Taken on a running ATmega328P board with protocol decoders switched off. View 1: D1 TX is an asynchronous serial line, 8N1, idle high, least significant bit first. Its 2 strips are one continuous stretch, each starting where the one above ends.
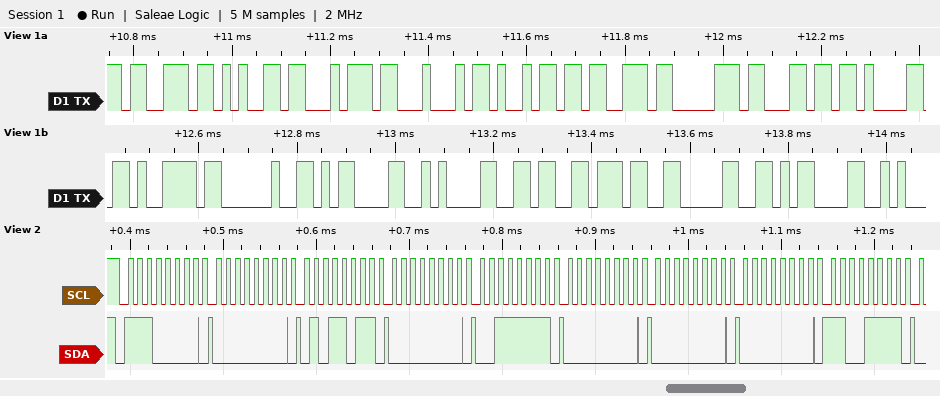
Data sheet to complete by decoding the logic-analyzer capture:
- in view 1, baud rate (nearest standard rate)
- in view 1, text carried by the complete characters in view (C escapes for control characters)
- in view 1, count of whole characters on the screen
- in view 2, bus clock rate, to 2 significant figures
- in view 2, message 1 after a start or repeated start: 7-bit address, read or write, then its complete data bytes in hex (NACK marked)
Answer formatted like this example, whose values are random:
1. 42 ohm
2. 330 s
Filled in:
1. 57600 baud
2. "setDisplay \r\n670\r"
3. 17
4. 100 kHz
5. 0x70 write: 00 5B 00 3F 00 00 00 CF
